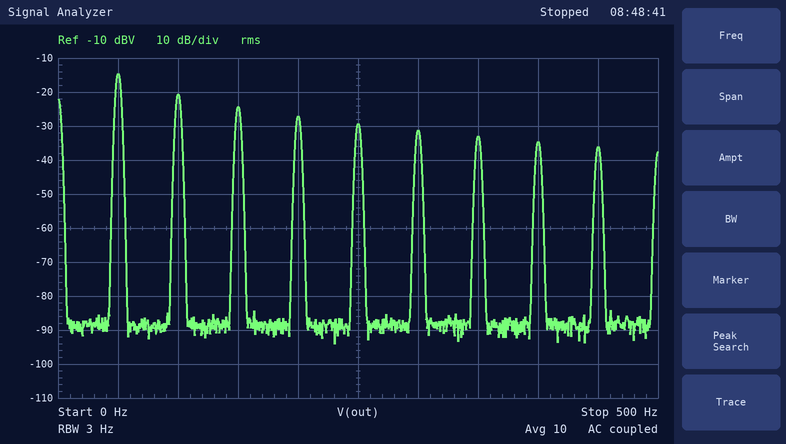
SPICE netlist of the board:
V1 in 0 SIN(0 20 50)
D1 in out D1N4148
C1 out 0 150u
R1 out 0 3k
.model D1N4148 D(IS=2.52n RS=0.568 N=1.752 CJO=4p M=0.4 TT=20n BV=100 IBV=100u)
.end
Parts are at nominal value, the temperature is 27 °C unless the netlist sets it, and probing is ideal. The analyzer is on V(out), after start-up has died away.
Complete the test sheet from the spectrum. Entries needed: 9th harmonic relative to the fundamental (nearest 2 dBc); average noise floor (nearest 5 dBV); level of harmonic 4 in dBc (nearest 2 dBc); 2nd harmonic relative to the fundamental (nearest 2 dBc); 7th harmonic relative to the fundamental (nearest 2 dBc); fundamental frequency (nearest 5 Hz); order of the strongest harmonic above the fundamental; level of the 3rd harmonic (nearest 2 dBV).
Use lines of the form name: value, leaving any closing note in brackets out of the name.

9th harmonic relative to the fundamental: -22 dBc
average noise floor: -90 dBV
level of harmonic 4 in dBc: -12 dBc
2nd harmonic relative to the fundamental: -6 dBc
7th harmonic relative to the fundamental: -18 dBc
fundamental frequency: 50 Hz
order of the strongest harmonic above the fundamental: 2
level of the 3rd harmonic: -24 dBV
